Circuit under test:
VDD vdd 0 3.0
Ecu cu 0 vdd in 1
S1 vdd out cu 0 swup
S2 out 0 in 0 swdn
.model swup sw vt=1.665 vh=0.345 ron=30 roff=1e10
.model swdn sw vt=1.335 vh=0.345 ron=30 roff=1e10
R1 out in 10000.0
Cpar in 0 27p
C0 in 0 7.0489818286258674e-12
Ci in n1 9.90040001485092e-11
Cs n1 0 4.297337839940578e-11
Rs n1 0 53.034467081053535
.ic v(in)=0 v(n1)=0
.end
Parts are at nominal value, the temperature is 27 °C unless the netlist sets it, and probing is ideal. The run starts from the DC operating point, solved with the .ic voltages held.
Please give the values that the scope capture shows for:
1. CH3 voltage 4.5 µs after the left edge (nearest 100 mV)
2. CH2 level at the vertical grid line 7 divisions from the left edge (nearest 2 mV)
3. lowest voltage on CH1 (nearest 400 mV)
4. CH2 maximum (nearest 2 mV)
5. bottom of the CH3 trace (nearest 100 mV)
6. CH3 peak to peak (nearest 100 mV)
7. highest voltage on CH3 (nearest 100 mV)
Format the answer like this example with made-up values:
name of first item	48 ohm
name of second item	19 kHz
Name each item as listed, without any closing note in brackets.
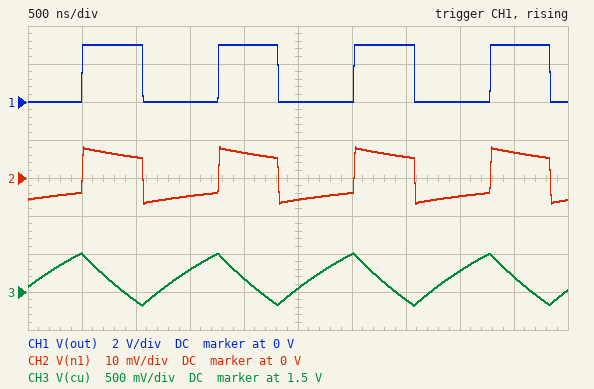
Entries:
CH3 voltage 4.5 µs after the left edge	1.7 V
CH2 level at the vertical grid line 7 divisions from the left edge	6 mV
lowest voltage on CH1	0 V
CH2 maximum	8 mV
bottom of the CH3 trace	1.3 V
CH3 peak to peak	700 mV
highest voltage on CH3	2.0 V
